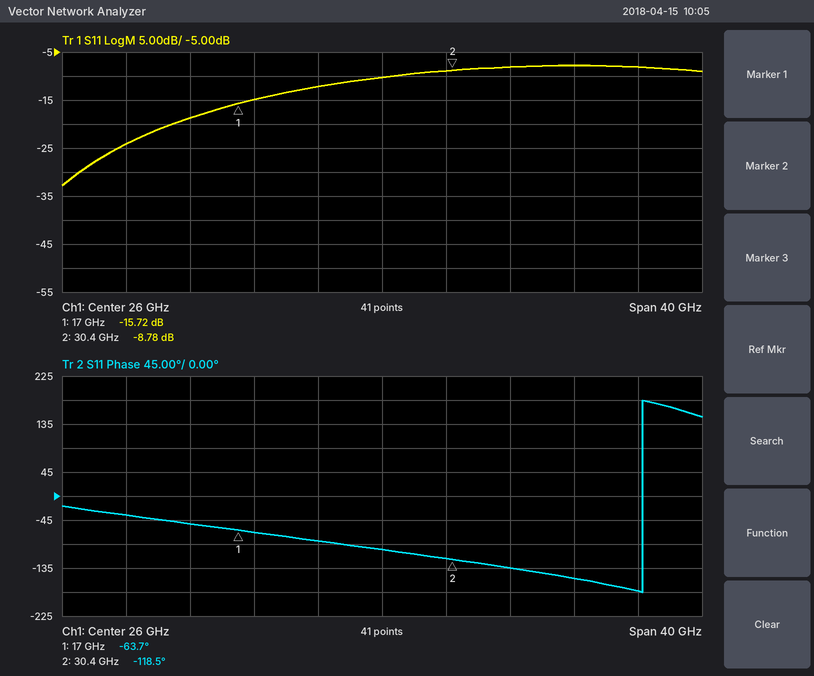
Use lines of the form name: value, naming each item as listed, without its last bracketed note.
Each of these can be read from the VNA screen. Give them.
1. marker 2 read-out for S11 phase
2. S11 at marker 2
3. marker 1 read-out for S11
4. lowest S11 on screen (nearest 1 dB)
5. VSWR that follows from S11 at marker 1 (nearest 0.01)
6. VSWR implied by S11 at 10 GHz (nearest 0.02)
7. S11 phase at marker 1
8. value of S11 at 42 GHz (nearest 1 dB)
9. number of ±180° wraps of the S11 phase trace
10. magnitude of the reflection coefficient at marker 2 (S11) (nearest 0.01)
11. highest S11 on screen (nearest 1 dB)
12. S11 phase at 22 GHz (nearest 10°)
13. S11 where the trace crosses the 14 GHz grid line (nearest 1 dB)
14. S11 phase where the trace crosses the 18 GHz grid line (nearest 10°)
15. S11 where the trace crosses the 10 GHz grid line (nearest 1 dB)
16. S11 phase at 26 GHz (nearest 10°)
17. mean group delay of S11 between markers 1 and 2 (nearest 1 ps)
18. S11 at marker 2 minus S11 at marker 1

marker 2 read-out for S11 phase: -118.5°
S11 at marker 2: -8.78 dB
marker 1 read-out for S11: -15.72 dB
lowest S11 on screen: -33 dB
VSWR that follows from S11 at marker 1: 1.39
VSWR implied by S11 at 10 GHz: 1.14
S11 phase at marker 1: -63.7°
value of S11 at 42 GHz: -8 dB
number of ±180° wraps of the S11 phase trace: 1
magnitude of the reflection coefficient at marker 2 (S11): 0.36
highest S11 on screen: -8 dB
S11 phase at 22 GHz: -80°
S11 where the trace crosses the 14 GHz grid line: -19 dB
S11 phase where the trace crosses the 18 GHz grid line: -70°
S11 where the trace crosses the 10 GHz grid line: -24 dB
S11 phase at 26 GHz: -100°
mean group delay of S11 between markers 1 and 2: 11 ps
S11 at marker 2 minus S11 at marker 1: 6.94 dB
